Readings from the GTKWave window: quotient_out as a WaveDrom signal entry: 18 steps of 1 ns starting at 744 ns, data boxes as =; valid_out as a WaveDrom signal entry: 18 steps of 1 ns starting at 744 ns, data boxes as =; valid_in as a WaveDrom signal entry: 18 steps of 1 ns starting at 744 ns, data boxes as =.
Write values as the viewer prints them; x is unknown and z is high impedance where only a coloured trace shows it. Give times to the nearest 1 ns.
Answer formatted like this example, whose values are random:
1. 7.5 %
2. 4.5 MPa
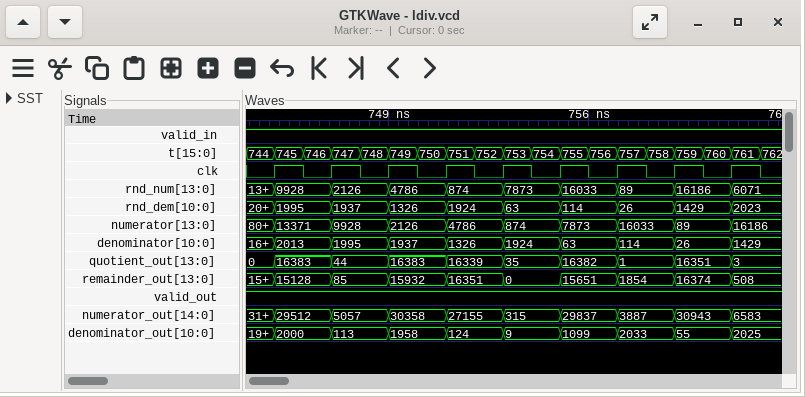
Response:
1. {name: 'quotient_out', wave: '==.=.=.=.=.=.=.=.=', data: '0 16383 44 16383 16339 35 16382 1 16351 3'}
2. {name: 'valid_out', wave: '1.................'}
3. {name: 'valid_in', wave: '1.................'}
